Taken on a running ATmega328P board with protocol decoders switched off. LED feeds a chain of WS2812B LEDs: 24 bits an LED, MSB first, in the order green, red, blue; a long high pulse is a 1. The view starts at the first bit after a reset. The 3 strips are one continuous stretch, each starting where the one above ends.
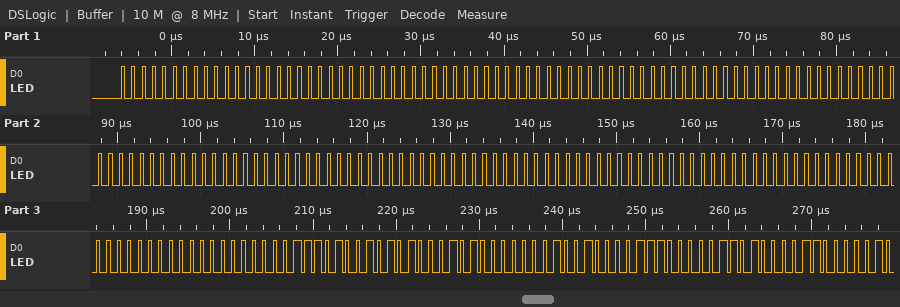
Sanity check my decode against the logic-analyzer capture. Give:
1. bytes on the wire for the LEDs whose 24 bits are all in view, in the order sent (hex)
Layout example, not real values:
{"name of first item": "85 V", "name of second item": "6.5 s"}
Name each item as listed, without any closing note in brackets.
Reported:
{"bytes on the wire for the LEDs whose 24 bits are all in view, in the order sent": "00 00 00 00 00 00 00 00 00 00 00 00 00 00 00 00 00 00 00 00 00 1D 2A 28 09 0E 0D"}
